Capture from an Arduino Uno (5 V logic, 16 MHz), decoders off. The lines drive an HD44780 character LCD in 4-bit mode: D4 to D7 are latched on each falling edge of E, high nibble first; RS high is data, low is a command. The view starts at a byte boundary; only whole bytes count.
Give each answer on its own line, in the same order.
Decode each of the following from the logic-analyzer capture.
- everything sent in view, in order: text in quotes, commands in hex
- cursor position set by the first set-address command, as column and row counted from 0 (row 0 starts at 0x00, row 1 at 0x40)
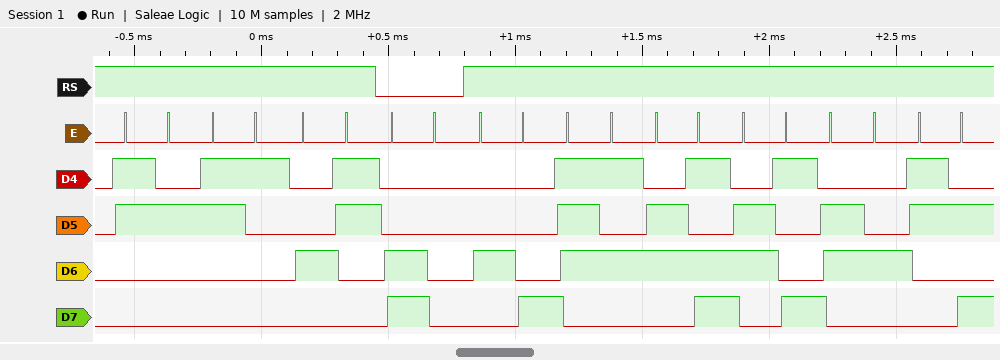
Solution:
"21C" 0xC0 "Humid:"
column 0, row 1
